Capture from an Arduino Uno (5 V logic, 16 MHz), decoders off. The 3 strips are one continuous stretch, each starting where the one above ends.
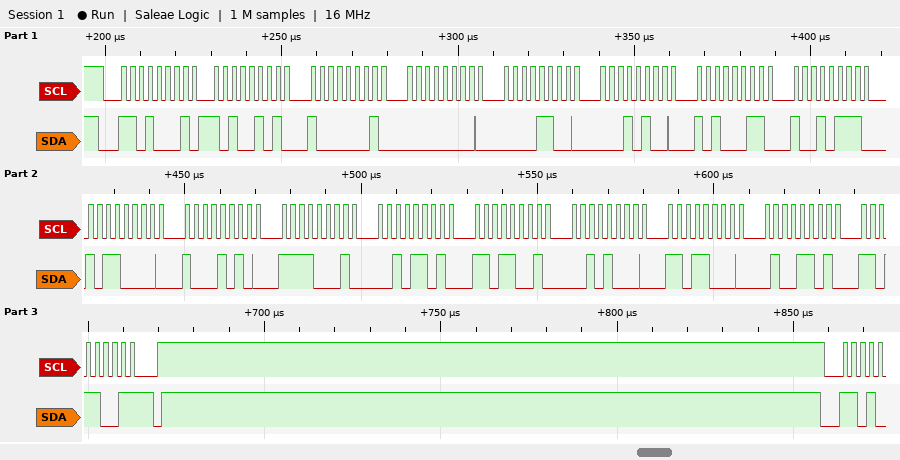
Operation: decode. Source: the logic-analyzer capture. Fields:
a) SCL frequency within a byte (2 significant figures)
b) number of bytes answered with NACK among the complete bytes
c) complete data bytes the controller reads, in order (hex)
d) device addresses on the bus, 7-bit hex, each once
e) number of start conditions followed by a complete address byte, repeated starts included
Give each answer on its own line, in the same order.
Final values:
400 kHz
1
A5 81 00 0C 14 A3 97 B0 8A F1 2D D9 28 D8 4D D9
0x68
1
